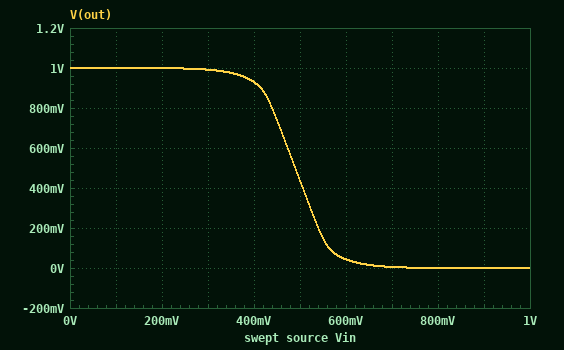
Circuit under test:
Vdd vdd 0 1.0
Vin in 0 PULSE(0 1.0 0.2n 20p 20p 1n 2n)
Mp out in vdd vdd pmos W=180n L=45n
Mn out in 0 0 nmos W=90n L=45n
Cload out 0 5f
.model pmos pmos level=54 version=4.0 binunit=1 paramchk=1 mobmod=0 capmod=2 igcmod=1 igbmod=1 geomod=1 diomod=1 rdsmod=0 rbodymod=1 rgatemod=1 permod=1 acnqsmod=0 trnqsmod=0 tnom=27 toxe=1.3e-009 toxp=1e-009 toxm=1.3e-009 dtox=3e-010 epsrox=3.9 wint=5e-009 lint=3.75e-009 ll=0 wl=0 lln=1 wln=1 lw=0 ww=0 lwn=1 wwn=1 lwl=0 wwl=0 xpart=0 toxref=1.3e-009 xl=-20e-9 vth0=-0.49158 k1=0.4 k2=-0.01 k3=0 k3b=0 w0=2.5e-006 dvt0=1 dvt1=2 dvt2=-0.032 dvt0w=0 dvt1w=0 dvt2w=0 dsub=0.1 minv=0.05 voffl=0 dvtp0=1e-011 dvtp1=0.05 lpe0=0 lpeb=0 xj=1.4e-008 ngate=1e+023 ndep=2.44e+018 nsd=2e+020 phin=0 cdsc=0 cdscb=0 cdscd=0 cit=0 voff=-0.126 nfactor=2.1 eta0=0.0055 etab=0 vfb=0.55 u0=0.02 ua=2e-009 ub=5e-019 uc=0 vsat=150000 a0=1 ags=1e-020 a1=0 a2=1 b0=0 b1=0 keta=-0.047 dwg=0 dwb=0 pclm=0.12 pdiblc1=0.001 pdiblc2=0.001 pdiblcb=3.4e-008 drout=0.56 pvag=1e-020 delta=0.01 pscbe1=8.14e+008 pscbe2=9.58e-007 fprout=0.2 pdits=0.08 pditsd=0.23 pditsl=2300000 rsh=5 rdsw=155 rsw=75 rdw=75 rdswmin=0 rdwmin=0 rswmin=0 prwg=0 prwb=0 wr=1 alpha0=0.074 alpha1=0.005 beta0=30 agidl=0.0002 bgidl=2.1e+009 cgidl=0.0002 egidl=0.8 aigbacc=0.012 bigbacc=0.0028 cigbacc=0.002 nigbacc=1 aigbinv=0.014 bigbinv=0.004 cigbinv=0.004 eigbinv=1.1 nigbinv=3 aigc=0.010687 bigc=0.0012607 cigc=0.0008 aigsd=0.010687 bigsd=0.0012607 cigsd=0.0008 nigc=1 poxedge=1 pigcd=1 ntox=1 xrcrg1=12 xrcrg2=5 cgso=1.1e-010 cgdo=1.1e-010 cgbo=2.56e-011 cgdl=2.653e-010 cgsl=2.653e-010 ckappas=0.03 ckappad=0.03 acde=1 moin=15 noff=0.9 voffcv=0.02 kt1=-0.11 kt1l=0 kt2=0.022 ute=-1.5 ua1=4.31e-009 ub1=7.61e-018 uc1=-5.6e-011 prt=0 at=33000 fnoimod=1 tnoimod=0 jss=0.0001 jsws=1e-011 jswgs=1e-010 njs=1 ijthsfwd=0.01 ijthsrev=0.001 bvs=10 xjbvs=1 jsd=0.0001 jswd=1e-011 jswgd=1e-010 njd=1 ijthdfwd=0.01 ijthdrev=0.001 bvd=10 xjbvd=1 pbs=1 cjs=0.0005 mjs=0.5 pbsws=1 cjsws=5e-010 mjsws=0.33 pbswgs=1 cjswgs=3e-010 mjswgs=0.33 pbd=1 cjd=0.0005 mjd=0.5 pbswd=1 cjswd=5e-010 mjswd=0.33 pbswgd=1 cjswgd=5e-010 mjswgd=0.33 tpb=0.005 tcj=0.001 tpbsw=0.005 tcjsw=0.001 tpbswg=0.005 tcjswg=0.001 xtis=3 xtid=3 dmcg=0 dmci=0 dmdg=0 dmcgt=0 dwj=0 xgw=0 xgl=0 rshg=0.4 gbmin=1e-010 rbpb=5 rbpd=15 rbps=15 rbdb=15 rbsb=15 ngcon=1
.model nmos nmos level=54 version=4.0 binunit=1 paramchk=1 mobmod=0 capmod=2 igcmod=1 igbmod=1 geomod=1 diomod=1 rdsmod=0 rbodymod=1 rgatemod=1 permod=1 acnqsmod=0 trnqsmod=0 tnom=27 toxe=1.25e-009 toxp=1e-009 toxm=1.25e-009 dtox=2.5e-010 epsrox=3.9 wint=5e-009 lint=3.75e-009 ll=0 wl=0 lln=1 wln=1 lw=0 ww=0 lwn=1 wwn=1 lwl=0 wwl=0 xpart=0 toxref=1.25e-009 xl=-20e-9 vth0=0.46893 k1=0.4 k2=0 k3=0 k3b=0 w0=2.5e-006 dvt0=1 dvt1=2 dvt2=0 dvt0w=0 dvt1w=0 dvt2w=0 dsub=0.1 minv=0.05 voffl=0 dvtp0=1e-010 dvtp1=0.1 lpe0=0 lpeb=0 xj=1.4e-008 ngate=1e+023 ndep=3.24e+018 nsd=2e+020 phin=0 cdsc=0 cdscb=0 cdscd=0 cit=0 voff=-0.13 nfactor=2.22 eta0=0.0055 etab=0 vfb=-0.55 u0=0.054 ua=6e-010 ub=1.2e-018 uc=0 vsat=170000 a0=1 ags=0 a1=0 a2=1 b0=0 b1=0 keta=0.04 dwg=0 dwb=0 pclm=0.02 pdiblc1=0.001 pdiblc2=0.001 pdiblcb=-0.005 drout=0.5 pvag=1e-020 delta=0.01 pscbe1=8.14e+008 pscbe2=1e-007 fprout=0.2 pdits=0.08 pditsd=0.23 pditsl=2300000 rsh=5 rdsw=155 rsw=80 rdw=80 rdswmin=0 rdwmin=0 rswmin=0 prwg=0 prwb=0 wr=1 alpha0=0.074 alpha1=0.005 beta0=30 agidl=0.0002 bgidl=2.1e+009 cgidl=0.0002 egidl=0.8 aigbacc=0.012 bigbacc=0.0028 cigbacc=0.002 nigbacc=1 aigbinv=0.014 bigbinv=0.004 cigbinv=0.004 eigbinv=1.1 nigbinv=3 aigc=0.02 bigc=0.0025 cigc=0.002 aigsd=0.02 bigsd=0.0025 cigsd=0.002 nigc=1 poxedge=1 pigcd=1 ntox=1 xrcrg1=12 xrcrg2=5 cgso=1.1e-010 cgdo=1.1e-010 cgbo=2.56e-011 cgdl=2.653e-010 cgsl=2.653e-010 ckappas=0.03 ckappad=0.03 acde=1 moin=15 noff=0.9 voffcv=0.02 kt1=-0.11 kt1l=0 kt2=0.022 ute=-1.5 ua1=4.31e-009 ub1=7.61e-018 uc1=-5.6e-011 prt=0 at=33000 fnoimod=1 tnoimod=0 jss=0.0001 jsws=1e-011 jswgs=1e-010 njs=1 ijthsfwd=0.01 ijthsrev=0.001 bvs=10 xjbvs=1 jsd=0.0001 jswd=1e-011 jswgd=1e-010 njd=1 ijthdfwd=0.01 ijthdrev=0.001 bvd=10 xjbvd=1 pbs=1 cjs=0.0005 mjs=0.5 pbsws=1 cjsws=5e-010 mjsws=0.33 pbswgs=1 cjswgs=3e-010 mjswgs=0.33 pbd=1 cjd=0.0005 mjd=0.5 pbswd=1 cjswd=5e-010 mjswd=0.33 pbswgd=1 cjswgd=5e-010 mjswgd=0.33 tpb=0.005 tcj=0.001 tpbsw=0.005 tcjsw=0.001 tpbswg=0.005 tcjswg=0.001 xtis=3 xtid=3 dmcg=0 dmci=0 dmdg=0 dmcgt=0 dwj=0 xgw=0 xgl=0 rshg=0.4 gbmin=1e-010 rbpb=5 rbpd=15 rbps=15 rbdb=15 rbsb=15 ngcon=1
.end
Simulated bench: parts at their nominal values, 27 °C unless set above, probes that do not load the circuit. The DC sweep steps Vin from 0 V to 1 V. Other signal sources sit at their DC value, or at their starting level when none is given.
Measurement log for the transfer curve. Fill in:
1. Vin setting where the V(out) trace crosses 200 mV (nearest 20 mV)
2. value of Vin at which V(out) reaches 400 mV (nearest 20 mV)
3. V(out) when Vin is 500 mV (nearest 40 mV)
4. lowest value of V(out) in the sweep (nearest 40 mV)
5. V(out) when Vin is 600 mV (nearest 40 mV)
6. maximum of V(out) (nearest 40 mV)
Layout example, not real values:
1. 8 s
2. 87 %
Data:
1. 540 mV
2. 500 mV
3. 440 mV
4. 0 V
5. 40 mV
6. 1.00 V
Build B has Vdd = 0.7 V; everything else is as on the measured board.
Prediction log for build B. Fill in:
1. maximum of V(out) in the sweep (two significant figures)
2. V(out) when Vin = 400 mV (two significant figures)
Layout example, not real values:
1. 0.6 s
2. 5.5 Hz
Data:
1. 700 mV
2. 17 mV
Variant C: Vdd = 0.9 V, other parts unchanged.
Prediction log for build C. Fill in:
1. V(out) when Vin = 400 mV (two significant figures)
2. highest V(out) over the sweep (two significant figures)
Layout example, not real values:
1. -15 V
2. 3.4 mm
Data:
1. 670 mV
2. 900 mV
